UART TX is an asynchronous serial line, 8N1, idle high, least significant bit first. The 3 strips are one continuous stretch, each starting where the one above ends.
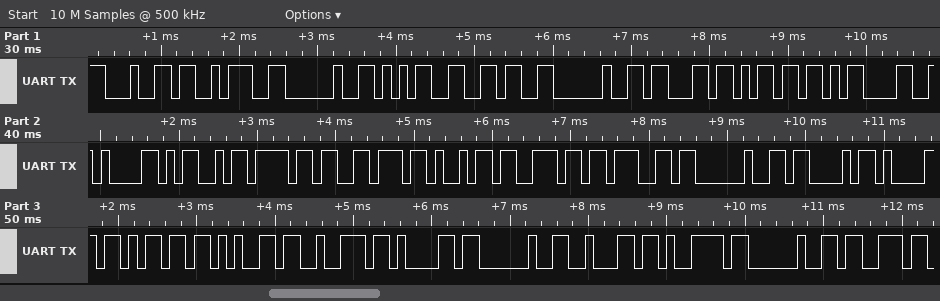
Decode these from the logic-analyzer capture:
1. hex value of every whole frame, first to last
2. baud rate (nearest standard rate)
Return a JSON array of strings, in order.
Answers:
["0x64 0x3A 0x20 0x35 0x36 0x20 0x63 0x6D 0x0D 0x0A 0x4D 0x6F 0x76 0x69 0x6E 0x67 0x20 0x43 0x61 0x6D 0x65 0x72 0x61 0x20 0x62 0x79 0x20 0x73", "9600 baud"]
